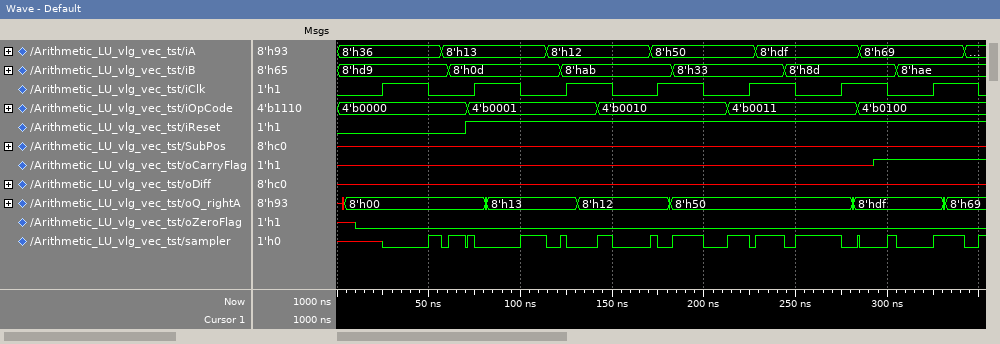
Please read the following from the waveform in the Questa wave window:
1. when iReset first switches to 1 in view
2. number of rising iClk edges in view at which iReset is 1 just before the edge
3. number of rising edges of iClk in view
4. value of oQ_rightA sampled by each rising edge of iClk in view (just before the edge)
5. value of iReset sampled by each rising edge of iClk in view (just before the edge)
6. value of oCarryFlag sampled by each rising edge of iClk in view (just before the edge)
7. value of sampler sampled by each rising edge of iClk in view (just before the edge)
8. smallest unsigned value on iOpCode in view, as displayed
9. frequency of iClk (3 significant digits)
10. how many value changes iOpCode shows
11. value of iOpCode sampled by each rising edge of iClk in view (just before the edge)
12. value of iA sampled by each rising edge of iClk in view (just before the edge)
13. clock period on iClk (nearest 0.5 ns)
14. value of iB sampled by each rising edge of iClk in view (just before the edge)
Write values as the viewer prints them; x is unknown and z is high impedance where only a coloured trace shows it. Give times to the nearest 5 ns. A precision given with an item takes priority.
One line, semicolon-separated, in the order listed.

70 ns; 6; 7; 8'h00, 8'h00, 8'h13, 8'h12, 8'h50, 8'h50, 8'hdf; 0 1 1 1 1 1 1; x x x x x x 1; x 1 1 1 1 1 0; 4'b0000; 20.0 MHz; 4; 4'b0000, 4'b0001, 4'b0001, 4'b0010, 4'b0011, 4'b0011, 4'b0100; 8'h36, 8'h13, 8'h12, 8'h50, 8'h50, 8'hdf, 8'h69; 50 ns; 8'hd9, 8'h0d, 8'hab, 8'hab, 8'h33, 8'h8d, 8'hae
